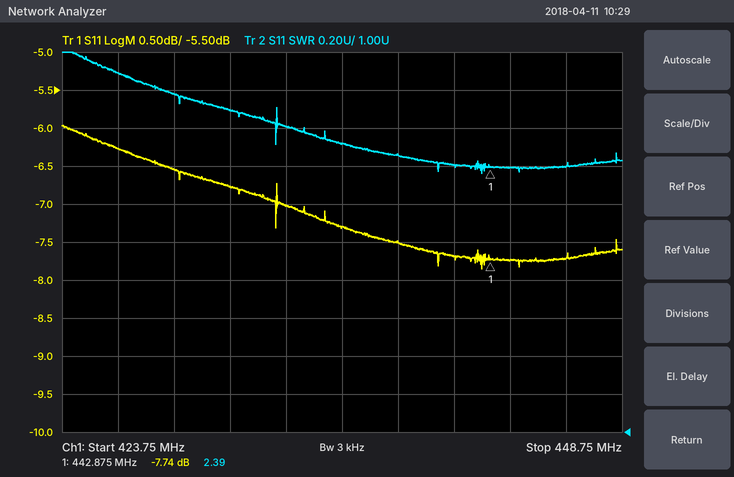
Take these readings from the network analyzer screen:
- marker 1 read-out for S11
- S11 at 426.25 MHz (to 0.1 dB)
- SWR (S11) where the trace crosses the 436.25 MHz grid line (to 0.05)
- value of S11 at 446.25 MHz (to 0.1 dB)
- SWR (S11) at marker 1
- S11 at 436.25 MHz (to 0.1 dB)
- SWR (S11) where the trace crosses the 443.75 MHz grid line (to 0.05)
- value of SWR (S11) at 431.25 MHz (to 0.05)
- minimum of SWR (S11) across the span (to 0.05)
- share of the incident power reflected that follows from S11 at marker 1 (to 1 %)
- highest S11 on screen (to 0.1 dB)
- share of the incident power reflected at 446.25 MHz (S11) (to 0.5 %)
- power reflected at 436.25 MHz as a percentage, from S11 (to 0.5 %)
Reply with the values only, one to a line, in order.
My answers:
-7.74 dB
-6.3 dB
2.50
-7.7 dB
2.39
-7.3 dB
2.40
2.70
2.35
17 %
-6.0 dB
17.0 %
18.5 %
